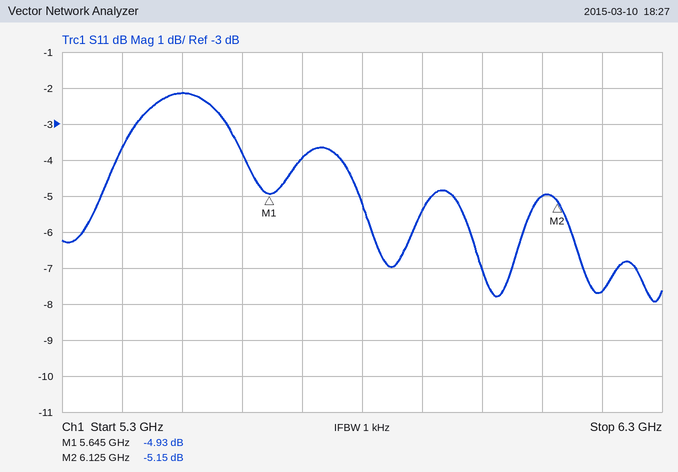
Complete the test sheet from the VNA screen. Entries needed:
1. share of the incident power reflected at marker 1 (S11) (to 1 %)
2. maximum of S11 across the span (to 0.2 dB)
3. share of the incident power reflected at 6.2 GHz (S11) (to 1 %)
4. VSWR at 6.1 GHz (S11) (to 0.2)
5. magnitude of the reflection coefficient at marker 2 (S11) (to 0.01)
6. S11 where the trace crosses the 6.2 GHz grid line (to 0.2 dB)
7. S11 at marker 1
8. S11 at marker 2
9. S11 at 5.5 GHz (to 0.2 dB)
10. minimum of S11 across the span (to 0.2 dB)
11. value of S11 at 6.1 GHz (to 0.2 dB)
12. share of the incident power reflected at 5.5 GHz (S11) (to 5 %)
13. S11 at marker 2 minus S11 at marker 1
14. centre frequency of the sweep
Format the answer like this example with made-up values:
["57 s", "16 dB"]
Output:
["32 %", "-2.2 dB", "17 %", "3.6", "0.55", "-7.6 dB", "-4.93 dB", "-5.15 dB", "-2.2 dB", "-8.0 dB", "-5.0 dB", "60 %", "-0.22 dB", "5.8 GHz"]
